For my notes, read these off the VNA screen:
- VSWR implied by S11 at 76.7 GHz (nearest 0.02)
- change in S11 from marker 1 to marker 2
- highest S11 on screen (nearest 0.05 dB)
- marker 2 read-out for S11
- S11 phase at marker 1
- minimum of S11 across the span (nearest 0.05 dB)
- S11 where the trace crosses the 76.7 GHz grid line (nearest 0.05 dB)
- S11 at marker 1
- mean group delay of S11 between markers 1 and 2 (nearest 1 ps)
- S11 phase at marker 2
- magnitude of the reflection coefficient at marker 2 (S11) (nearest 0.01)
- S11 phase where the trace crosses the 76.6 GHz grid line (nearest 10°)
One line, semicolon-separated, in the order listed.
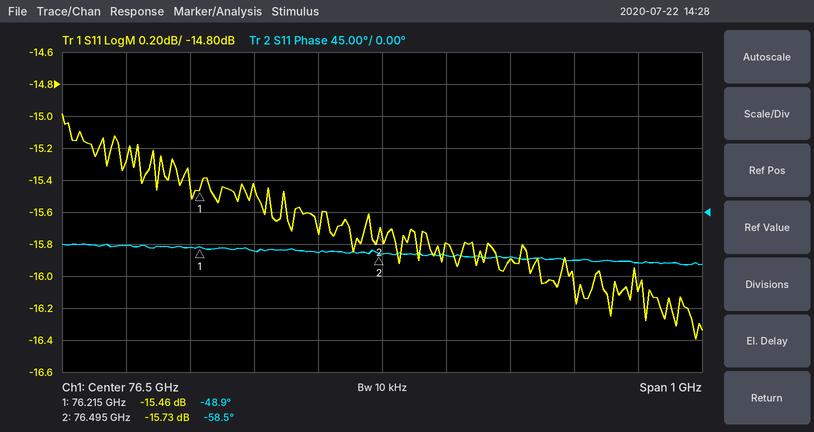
1.38; -0.27 dB; -15.00 dB; -15.73 dB; -48.9°; -16.40 dB; -15.90 dB; -15.46 dB; 95 ps; -58.5°; 0.16; -60°
